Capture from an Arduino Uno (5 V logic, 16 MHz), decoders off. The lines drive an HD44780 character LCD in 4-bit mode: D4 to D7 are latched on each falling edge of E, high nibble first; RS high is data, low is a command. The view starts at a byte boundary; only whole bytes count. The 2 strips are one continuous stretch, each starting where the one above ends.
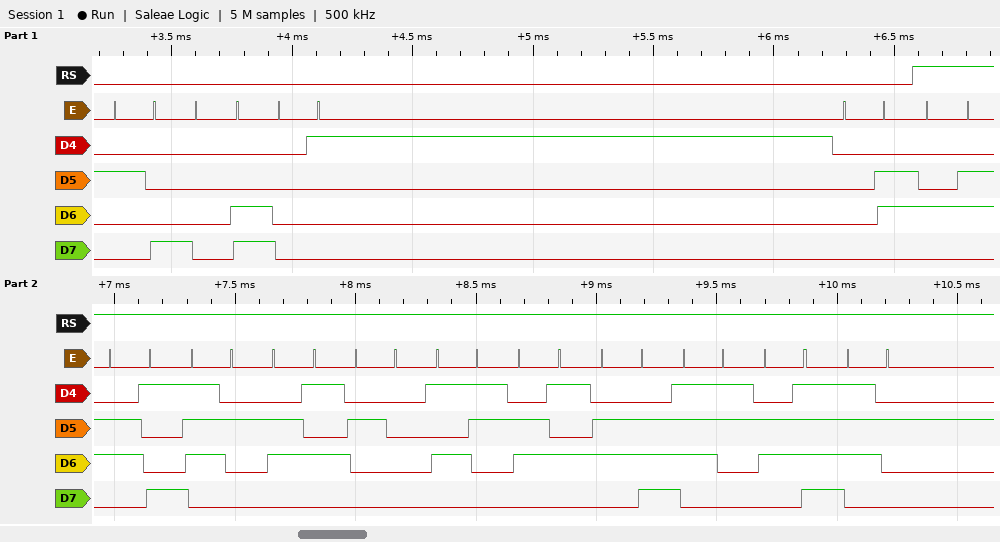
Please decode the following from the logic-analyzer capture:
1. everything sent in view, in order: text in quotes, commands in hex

0x28 0x0C 0x01 0x06 "Fire Sensor"
